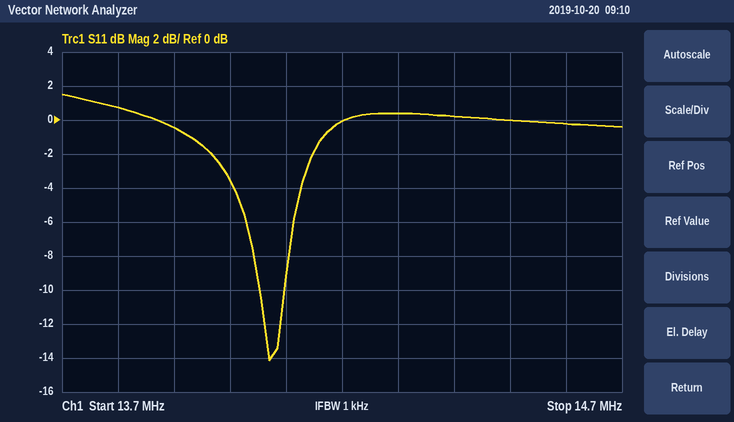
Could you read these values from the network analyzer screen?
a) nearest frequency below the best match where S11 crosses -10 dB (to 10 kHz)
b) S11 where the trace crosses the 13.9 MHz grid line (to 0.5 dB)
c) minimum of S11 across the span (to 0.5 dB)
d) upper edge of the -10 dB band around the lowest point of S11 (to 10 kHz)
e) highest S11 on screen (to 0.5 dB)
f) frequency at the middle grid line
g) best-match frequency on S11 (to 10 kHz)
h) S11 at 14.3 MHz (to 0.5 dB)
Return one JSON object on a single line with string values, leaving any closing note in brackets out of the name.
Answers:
{"nearest frequency below the best match where S11 crosses -10 dB": "14.05 MHz", "S11 where the trace crosses the 13.9 MHz grid line": "-0.5 dB", "minimum of S11 across the span": "-14.0 dB", "upper edge of the -10 dB band around the lowest point of S11": "14.10 MHz", "highest S11 on screen": "1.5 dB", "frequency at the middle grid line": "14.2 MHz", "best-match frequency on S11": "14.07 MHz", "S11 at 14.3 MHz": "0.5 dB"}
